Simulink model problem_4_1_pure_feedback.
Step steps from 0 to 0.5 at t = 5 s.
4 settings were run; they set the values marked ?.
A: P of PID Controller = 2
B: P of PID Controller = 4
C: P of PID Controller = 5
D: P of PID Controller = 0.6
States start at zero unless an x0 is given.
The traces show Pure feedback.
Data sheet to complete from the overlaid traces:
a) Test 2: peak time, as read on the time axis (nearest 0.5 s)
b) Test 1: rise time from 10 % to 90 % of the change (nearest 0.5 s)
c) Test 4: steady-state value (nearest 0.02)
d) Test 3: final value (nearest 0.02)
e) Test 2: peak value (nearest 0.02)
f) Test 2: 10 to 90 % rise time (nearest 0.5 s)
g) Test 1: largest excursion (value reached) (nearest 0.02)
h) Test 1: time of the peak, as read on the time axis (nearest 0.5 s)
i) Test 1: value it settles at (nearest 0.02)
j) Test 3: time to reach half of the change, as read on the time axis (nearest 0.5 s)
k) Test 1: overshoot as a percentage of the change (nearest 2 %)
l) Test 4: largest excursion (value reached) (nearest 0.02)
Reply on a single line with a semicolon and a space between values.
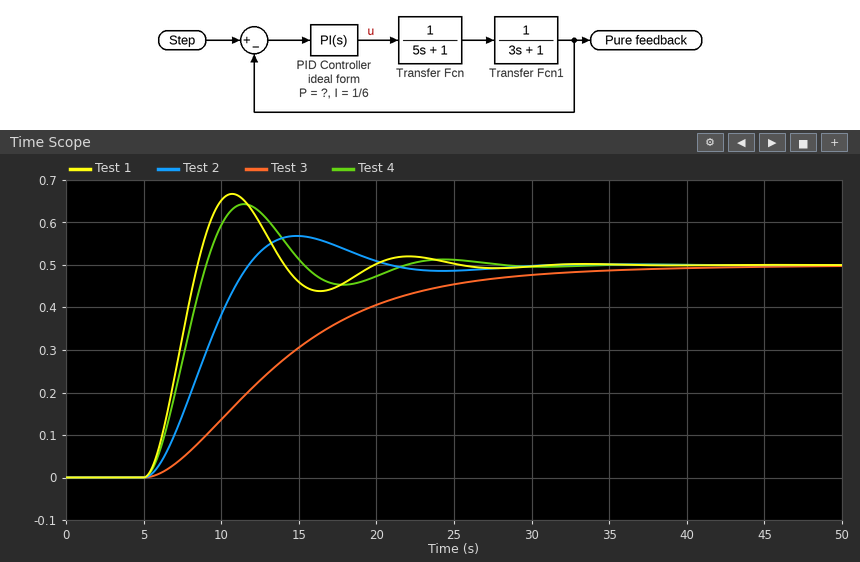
15.0 s; 2.5 s; 0.50; 0.50; 0.56; 4.5 s; 0.66; 10.5 s; 0.50; 13.0 s; 34 %; 0.64
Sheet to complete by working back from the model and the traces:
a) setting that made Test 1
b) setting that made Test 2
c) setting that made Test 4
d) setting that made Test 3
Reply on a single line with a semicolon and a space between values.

C; A; B; D
